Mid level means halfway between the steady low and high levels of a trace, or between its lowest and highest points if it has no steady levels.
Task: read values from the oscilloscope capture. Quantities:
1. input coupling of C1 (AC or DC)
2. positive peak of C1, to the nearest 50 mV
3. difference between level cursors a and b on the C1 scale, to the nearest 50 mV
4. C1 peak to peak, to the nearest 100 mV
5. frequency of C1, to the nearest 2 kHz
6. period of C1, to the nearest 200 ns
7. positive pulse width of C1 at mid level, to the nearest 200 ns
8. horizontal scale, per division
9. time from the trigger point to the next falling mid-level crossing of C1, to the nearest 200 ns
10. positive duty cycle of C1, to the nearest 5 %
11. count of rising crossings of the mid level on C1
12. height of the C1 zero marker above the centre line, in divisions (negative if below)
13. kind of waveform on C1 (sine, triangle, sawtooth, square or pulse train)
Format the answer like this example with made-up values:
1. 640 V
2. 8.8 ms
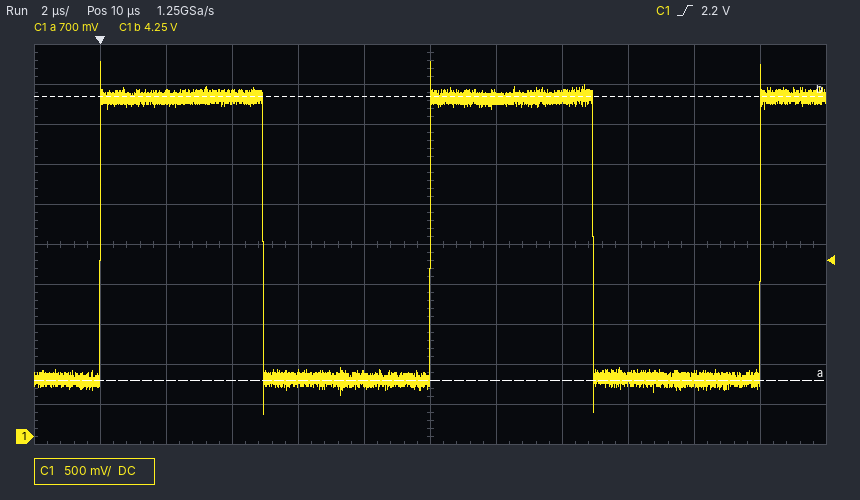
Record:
1. DC
2. 4.70 V
3. 3.55 V
4. 4.40 V
5. 100 kHz
6. 10.0 µs
7. 5.0 µs
8. 2 µs
9. 5.0 µs
10. 50 %
11. 3
12. -4.8 div
13. square
